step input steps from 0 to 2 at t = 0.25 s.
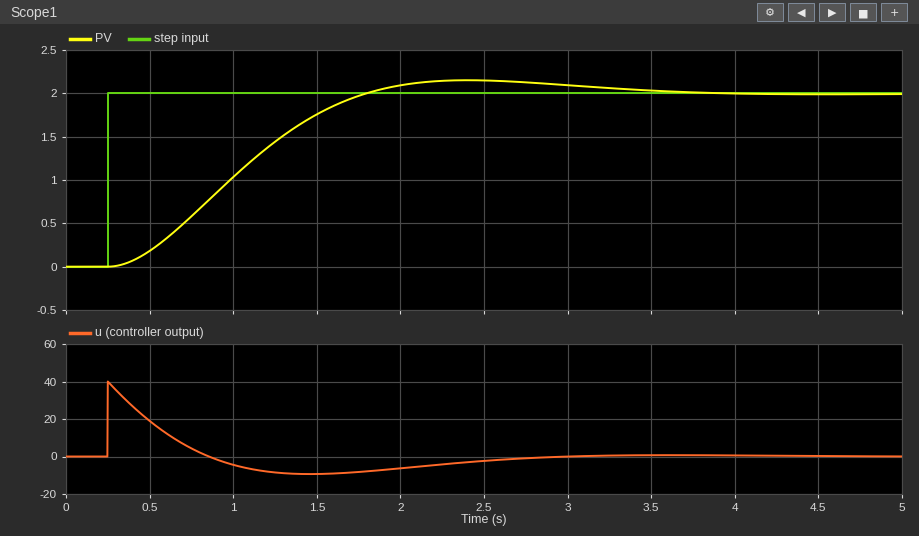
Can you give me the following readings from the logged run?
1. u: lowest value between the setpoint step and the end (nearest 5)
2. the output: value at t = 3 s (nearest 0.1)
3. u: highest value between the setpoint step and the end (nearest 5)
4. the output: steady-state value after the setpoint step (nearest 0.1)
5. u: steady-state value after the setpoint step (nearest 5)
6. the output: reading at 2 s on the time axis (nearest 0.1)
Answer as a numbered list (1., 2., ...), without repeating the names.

1. -10
2. 2.1
3. 40
4. 2.0
5. 0
6. 2.1
